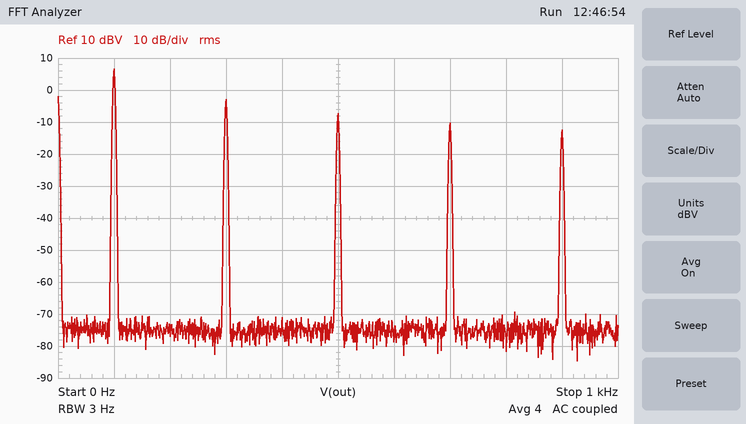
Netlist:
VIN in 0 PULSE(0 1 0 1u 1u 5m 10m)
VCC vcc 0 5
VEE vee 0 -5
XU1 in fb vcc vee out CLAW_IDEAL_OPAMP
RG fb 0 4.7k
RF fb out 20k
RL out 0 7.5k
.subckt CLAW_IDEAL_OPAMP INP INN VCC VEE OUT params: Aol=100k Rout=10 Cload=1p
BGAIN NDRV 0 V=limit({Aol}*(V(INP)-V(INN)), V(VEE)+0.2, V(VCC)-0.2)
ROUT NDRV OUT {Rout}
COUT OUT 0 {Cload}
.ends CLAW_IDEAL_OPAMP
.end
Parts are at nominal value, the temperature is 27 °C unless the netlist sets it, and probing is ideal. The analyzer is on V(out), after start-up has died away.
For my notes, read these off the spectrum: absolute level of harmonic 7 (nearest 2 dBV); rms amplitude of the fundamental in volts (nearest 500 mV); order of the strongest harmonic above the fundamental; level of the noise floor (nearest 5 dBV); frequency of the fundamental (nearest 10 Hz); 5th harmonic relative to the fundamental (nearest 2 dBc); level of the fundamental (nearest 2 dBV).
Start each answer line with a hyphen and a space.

- -10 dBV
- 2.0 V
- 3
- -75 dBV
- 100 Hz
- -14 dBc
- 6 dBV
